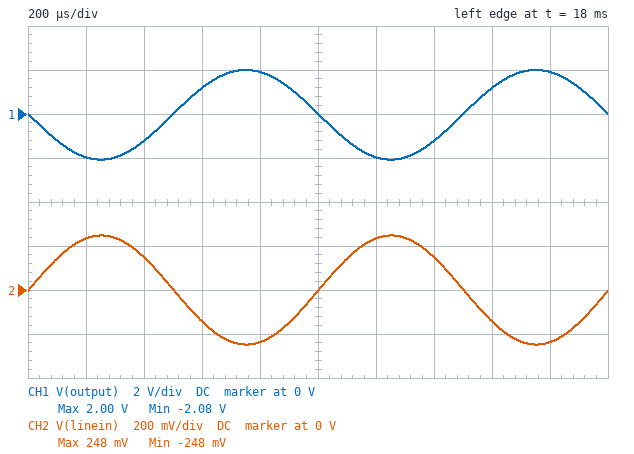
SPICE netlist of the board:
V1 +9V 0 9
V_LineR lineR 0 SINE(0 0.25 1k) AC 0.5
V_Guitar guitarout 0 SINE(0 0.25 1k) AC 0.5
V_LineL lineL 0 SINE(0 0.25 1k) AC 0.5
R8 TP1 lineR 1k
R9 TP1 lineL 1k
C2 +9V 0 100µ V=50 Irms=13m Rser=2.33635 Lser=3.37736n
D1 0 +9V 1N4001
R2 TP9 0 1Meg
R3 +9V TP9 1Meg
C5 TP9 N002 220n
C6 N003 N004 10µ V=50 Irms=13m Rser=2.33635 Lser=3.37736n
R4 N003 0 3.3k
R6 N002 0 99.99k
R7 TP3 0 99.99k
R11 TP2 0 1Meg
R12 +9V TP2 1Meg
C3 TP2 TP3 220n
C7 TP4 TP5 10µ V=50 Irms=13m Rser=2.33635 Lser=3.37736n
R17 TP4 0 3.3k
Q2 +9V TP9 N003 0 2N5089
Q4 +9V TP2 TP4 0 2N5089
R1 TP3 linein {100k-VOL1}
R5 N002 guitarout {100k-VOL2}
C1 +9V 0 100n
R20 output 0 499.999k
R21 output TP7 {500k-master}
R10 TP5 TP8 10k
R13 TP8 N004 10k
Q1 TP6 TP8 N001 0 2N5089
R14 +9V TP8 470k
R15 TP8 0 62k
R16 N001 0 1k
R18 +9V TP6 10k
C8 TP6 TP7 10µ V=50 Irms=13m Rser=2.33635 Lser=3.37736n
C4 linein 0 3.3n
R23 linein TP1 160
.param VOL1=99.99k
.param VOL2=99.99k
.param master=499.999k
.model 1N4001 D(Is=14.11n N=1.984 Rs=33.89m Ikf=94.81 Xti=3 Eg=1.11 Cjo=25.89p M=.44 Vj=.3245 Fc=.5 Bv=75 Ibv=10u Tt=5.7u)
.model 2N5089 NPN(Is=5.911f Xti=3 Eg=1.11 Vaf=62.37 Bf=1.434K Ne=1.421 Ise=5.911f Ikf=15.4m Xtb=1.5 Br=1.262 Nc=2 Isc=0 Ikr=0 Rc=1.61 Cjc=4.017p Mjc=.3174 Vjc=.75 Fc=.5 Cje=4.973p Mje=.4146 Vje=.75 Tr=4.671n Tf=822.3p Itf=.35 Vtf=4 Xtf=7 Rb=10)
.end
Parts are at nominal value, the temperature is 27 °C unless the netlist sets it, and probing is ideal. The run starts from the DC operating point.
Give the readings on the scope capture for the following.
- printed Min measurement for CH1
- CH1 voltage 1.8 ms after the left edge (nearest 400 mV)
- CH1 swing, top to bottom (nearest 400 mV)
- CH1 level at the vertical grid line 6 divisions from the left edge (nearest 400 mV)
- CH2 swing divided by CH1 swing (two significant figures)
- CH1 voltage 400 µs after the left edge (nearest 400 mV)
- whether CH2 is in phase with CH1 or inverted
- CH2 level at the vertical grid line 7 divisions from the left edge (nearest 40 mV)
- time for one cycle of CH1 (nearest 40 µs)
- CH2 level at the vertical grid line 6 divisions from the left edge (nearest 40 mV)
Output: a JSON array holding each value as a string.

["-2.08 V", "2.0 V", "4.0 V", "-2.0 V", "0.12", "-1.2 V", "inverted", "160 mV", "1.00 ms", "240 mV"]
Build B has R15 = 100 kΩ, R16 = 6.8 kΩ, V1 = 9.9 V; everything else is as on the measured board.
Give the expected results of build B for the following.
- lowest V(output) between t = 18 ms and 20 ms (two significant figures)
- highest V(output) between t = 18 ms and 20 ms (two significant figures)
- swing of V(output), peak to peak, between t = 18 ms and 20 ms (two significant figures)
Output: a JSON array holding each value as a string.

["-330 mV", "330 mV", "650 mV"]
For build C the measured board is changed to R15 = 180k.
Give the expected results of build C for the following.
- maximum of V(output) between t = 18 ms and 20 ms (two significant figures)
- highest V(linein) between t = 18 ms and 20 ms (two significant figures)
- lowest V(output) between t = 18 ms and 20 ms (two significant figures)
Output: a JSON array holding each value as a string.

["1.9 V", "250 mV", "-15 mV"]
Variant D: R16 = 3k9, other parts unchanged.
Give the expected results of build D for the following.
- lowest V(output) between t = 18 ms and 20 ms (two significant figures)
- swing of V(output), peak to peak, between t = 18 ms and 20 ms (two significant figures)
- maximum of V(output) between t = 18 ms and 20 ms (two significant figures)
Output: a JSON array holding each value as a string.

["-540 mV", "1.1 V", "520 mV"]
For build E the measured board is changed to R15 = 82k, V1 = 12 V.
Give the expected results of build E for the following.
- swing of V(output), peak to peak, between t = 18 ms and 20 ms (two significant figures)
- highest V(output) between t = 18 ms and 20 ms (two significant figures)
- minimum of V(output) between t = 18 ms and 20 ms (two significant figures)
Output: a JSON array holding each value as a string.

["2.8 V", "2.2 V", "-570 mV"]
